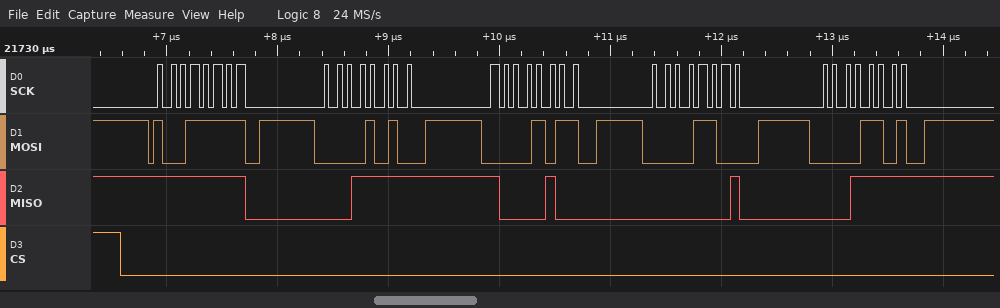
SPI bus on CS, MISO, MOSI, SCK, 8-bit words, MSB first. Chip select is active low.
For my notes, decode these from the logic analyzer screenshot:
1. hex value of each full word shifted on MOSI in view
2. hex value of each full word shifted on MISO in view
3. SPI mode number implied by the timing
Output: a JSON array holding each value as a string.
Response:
["9F, 0A, 0B, 0C, 0D", "FF, 1F, 84, 01, 1F", "0"]
